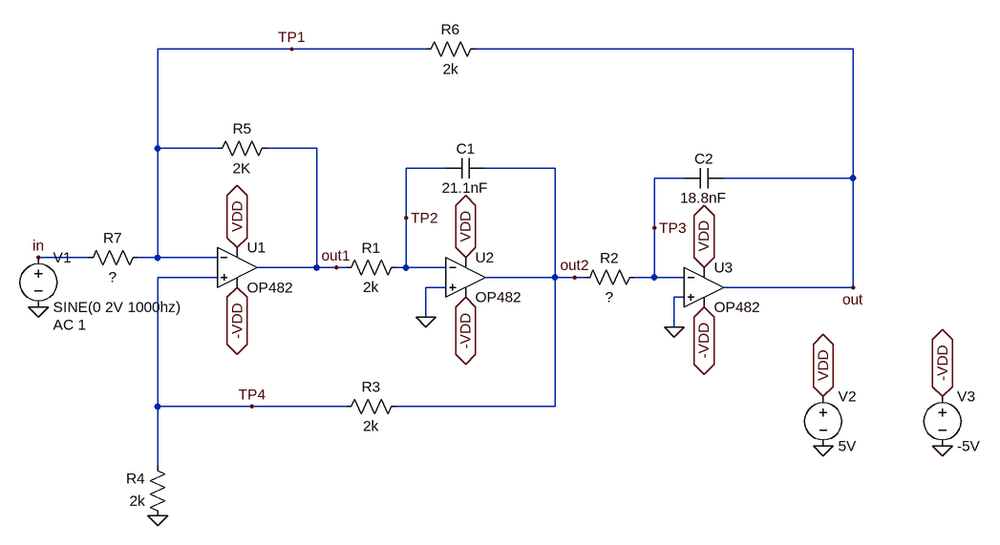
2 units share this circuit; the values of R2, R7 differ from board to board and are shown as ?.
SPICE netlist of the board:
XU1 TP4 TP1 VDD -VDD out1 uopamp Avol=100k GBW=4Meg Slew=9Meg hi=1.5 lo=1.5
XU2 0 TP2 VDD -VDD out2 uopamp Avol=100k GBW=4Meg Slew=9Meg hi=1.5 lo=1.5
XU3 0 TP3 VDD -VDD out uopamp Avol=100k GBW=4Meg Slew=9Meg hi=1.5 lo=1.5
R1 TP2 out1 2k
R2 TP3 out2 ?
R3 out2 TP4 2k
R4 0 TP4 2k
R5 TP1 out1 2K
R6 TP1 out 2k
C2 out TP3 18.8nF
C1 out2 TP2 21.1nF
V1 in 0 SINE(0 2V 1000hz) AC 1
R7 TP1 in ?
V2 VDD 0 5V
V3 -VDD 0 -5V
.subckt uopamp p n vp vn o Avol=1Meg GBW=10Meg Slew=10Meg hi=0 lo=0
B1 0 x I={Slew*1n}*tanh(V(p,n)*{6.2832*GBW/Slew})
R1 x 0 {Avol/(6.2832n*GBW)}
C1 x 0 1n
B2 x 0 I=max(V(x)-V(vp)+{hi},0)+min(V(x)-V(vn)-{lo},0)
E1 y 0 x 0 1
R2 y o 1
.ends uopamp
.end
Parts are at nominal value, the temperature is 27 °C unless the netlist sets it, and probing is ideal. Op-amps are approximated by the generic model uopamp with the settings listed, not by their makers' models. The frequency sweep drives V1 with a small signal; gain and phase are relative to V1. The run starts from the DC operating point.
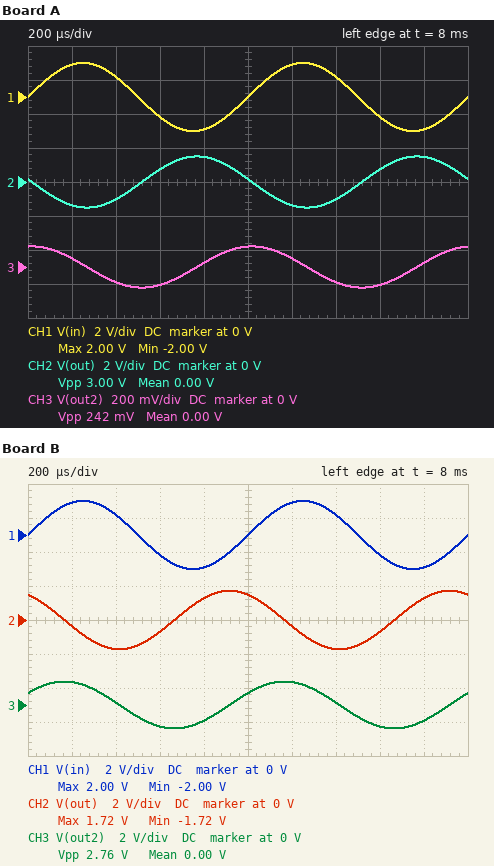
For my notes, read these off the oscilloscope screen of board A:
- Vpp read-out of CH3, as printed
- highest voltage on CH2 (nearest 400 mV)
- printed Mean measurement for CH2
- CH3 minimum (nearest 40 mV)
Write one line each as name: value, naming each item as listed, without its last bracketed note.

Vpp read-out of CH3, as printed: 242 mV
highest voltage on CH2: 1.6 V
printed Mean measurement for CH2: 0.00 V
CH3 minimum: -120 mV
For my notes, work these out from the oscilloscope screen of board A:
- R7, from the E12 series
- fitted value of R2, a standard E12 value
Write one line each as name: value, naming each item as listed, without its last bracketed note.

R7, from the E12 series: 2.7 kΩ
fitted value of R2, a standard E12 value: 680 Ω
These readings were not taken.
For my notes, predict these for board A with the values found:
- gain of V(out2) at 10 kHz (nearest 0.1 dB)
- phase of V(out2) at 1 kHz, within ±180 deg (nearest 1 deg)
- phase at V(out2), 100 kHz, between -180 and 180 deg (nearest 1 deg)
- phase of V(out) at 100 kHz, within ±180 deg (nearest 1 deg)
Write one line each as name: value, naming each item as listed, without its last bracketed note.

gain of V(out2) at 10 kHz: -8.4 dB
phase of V(out2) at 1 kHz, within ±180 deg: 84 deg
phase at V(out2), 100 kHz, between -180 and 180 deg: -92 deg
phase of V(out) at 100 kHz, within ±180 deg: -4 deg
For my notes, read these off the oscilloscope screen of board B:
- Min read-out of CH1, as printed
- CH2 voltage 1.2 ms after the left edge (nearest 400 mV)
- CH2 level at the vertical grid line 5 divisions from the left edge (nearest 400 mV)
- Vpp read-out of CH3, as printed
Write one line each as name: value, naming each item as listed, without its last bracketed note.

Min read-out of CH1, as printed: -2.00 V
CH2 voltage 1.2 ms after the left edge: -400 mV
CH2 level at the vertical grid line 5 divisions from the left edge: 1.6 V
Vpp read-out of CH3, as printed: 2.76 V
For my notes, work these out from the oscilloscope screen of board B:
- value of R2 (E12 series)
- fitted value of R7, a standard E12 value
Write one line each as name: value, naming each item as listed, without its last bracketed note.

value of R2: 6.8 kΩ
fitted value of R7, a standard E12 value: 1.5 kΩ
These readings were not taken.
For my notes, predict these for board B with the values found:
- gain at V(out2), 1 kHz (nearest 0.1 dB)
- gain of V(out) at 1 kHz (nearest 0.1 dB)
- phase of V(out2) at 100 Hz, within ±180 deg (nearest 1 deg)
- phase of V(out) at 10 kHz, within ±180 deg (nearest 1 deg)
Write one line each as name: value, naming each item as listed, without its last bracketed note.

gain at V(out2), 1 kHz: -3.2 dB
gain of V(out) at 1 kHz: -1.3 dB
phase of V(out2) at 100 Hz, within ±180 deg: 82 deg
phase of V(out) at 10 kHz, within ±180 deg: 33 deg
